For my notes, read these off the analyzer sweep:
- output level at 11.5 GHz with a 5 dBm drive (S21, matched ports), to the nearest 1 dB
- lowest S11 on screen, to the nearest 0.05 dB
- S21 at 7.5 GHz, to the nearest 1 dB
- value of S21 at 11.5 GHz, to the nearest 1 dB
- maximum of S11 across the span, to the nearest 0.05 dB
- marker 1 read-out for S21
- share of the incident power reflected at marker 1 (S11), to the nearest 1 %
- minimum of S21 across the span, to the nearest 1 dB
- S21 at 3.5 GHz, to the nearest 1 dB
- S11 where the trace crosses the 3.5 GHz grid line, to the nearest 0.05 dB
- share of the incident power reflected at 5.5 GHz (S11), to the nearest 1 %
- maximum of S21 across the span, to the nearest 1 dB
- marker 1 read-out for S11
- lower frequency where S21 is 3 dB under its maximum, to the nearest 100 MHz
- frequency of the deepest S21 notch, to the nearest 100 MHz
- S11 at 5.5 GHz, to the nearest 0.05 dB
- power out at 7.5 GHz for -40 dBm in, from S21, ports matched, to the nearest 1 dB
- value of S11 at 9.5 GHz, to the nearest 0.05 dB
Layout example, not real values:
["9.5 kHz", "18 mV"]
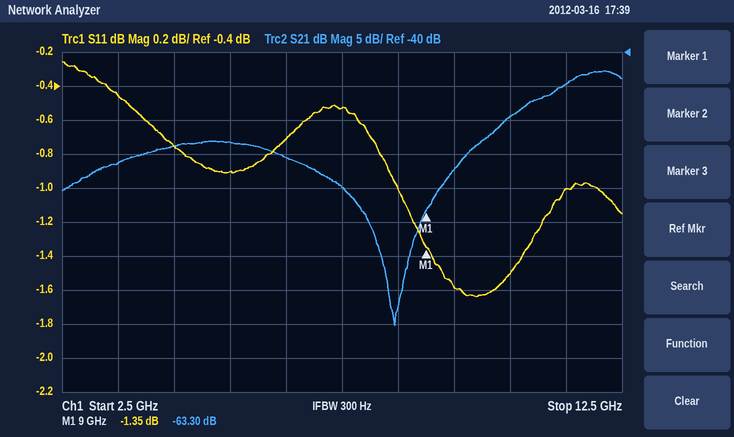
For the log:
["-40 dBm", "-1.65 dB", "-60 dB", "-45 dB", "-0.25 dB", "-63.30 dB", "73 %", "-80 dB", "-56 dB", "-0.45 dB", "81 %", "-43 dB", "-1.35 dB", "11.3 GHz", "8.4 GHz", "-0.90 dB", "-100 dBm", "-1.60 dB"]
